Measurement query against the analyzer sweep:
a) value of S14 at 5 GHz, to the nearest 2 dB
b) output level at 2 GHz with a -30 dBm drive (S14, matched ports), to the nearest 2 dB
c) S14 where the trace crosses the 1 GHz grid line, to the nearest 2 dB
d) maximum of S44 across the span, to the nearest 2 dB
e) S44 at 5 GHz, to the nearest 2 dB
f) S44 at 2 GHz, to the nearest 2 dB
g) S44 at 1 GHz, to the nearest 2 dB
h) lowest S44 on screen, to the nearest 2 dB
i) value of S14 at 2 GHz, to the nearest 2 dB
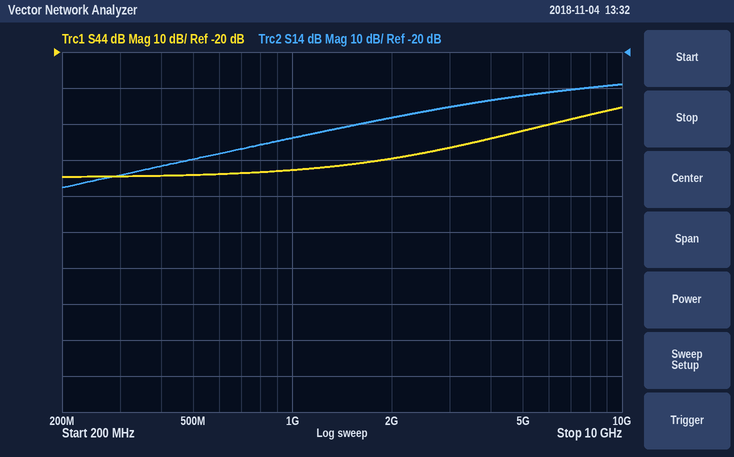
-32 dB
-68 dBm
-44 dB
-36 dB
-42 dB
-50 dB
-52 dB
-54 dB
-38 dB
